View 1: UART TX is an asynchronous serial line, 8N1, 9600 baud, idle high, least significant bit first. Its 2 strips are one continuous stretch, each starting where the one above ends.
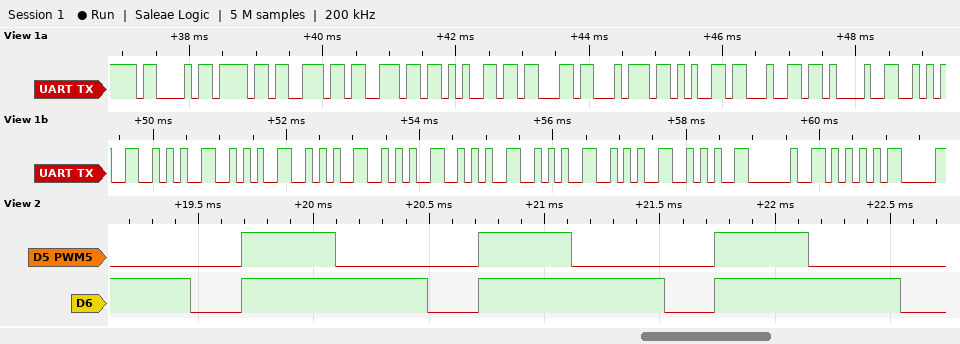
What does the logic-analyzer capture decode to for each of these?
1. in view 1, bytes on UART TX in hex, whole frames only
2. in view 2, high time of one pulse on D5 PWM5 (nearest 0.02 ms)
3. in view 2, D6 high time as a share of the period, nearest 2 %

0x43 0x6F 0x6E 0x6E 0x65 0x63 0x74 0x65 0x64 0x21 0x2A 0x2A 0x2A 0x2A 0x2A 0x2A 0x2A 0x2A 0x2A 0x20 0x55
0.40 ms
78 %
